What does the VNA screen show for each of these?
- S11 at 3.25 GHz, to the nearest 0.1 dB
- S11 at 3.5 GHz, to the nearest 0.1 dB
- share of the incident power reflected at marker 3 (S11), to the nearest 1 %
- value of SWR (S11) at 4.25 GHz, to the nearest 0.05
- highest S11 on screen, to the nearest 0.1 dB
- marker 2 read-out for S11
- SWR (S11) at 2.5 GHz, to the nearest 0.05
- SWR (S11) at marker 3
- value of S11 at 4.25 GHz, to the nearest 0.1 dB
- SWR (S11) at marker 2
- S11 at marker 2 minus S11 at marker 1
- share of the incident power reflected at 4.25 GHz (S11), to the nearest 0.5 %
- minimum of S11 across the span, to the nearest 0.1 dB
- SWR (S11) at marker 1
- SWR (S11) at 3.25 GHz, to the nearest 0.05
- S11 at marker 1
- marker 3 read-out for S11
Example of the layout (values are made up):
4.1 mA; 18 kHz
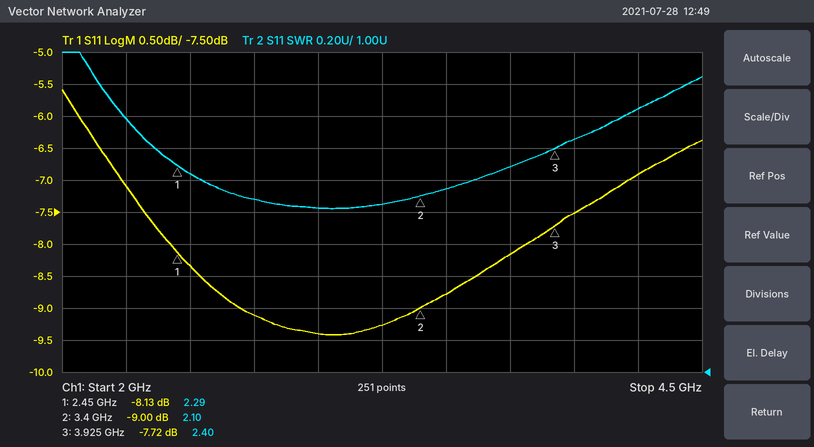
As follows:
-9.3 dB; -8.8 dB; 17 %; 2.65; -5.6 dB; -9.00 dB; 2.25; 2.40; -6.9 dB; 2.10; -0.87 dB; 20.5 %; -9.4 dB; 2.29; 2.05; -8.13 dB; -7.72 dB
